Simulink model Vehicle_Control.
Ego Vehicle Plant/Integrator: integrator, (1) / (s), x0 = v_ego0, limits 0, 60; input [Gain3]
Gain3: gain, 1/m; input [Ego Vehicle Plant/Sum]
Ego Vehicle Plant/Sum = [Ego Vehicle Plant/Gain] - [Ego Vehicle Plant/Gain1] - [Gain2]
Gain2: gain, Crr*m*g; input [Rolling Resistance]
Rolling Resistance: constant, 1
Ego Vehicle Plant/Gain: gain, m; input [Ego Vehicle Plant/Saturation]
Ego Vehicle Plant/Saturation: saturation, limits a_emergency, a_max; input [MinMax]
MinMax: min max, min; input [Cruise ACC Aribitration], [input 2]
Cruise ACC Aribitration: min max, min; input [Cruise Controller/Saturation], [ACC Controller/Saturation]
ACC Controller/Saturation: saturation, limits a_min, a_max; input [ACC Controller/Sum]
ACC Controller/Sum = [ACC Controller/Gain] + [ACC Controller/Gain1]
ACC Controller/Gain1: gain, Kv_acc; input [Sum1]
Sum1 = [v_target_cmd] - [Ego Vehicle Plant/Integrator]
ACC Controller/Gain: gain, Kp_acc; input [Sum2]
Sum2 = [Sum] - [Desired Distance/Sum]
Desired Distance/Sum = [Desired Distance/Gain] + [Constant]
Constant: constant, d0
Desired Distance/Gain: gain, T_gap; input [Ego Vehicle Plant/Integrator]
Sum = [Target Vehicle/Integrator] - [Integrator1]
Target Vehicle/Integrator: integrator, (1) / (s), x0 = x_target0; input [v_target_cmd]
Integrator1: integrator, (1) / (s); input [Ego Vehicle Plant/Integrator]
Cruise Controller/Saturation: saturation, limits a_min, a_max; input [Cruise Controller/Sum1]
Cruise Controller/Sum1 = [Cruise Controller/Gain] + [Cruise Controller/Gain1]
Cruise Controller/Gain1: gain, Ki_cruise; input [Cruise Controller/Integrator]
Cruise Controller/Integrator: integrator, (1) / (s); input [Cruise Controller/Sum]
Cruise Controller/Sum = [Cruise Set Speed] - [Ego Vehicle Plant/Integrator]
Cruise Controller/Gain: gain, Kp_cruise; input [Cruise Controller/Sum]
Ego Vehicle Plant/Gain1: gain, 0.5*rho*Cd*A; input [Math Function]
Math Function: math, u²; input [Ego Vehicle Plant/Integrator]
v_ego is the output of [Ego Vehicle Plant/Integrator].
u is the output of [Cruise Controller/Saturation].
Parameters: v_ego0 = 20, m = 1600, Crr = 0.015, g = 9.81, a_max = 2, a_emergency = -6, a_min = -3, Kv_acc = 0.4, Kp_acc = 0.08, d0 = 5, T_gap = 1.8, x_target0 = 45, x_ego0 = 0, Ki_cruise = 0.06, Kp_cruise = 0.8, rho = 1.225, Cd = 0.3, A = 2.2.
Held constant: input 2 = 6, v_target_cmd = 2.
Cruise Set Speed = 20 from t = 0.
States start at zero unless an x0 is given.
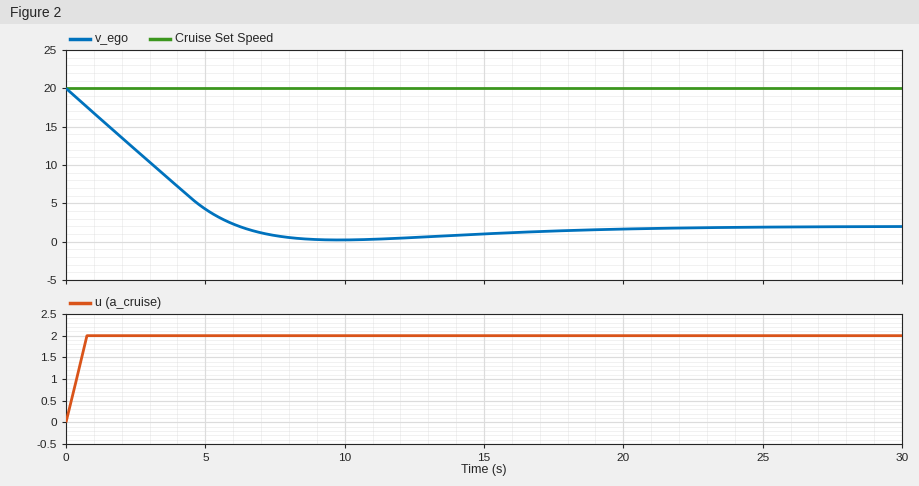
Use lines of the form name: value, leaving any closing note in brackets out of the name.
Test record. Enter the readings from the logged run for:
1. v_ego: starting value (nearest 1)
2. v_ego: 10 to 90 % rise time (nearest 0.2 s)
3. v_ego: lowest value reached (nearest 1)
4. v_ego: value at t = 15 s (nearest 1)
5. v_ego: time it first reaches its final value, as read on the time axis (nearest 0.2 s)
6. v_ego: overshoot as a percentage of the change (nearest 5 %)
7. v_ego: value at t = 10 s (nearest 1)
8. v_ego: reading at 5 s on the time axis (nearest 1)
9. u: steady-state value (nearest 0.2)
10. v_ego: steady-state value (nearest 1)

v_ego: starting value: 20
v_ego: 10 to 90 % rise time: 4.6 s
v_ego: lowest value reached: 0
v_ego: value at t = 15 s: 1
v_ego: time it first reaches its final value, as read on the time axis: 6.2 s
v_ego: overshoot as a percentage of the change: 10 %
v_ego: value at t = 10 s: 0
v_ego: reading at 5 s on the time axis: 4
u: steady-state value: 2.0
v_ego: steady-state value: 2
